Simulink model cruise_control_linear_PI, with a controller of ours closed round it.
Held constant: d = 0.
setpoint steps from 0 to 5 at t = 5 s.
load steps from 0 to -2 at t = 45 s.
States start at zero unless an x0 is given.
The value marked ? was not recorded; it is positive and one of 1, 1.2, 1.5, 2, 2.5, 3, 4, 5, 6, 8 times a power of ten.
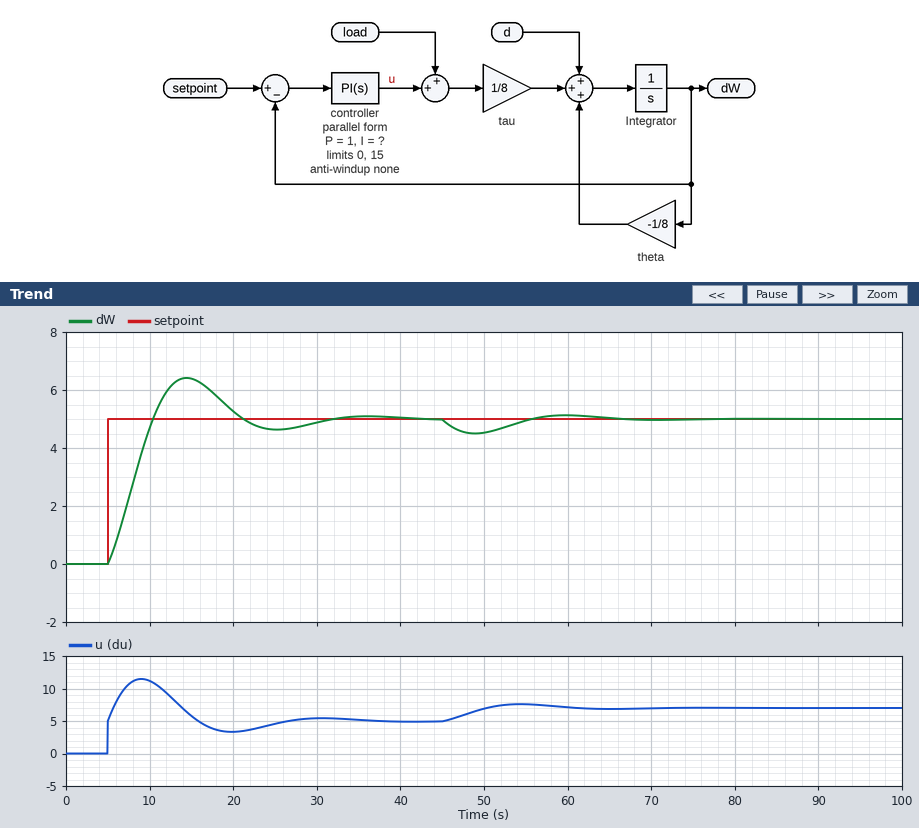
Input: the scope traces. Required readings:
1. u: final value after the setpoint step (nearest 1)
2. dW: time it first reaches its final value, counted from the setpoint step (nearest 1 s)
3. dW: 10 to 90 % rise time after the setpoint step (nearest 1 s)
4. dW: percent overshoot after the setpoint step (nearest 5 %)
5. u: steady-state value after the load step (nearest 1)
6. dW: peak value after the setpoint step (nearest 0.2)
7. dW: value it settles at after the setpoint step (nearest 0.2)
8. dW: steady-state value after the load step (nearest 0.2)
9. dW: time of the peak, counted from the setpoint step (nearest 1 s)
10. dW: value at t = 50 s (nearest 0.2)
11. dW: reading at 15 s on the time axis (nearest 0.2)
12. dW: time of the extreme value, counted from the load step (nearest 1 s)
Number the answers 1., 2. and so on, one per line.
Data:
1. 5
2. 5 s
3. 4 s
4. 30 %
5. 7
6. 6.4
7. 5.0
8. 5.0
9. 9 s
10. 4.6
11. 6.4
12. 4 s
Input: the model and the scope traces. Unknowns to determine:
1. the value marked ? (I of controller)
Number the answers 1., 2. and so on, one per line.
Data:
1. 0.8
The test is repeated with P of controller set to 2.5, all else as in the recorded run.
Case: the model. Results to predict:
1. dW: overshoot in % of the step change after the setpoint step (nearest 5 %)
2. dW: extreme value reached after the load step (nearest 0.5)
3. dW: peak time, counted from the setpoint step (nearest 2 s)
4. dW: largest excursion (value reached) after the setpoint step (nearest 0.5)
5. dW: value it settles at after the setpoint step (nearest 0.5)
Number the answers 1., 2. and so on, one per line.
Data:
1. 10 %
2. 4.5
3. 8 s
4. 5.5
5. 5.0
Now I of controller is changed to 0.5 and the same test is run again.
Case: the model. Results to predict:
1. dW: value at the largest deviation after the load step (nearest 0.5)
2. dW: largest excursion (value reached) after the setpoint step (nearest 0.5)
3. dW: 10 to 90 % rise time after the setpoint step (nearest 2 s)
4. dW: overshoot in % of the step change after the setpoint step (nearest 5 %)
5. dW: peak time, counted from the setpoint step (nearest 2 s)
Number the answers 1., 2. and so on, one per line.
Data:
1. 4.5
2. 6.0
3. 6 s
4. 20 %
5. 12 s
